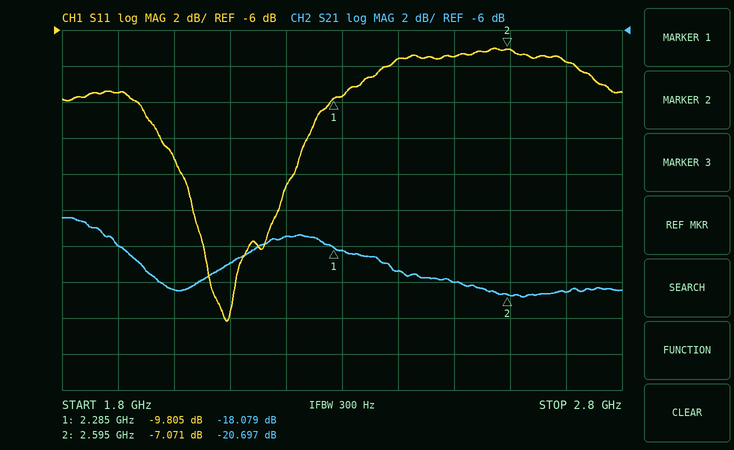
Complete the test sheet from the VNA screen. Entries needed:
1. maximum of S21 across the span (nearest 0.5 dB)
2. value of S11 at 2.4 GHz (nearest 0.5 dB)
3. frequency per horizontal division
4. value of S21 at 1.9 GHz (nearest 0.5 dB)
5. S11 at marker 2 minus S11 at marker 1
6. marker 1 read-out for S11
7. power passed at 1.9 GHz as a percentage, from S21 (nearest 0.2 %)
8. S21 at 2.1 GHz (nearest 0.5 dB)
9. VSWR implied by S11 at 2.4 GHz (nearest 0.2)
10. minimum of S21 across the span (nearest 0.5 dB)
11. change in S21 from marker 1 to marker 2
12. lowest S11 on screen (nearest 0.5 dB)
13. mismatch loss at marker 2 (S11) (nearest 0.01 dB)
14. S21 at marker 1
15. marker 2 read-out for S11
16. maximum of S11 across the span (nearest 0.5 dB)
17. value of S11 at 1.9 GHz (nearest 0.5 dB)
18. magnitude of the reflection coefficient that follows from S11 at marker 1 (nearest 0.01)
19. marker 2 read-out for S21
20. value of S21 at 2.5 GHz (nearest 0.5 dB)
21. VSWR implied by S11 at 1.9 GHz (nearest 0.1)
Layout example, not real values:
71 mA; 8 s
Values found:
-16.5 dB; -7.5 dB; 100 MHz; -18.0 dB; 2.734 dB; -9.805 dB; 1.6 %; -19.0 dB; 2.4; -21.0 dB; -2.618 dB; -22.0 dB; 0.95 dB; -18.079 dB; -7.071 dB; -7.0 dB; -9.5 dB; 0.32; -20.697 dB; -20.0 dB; 2.0
